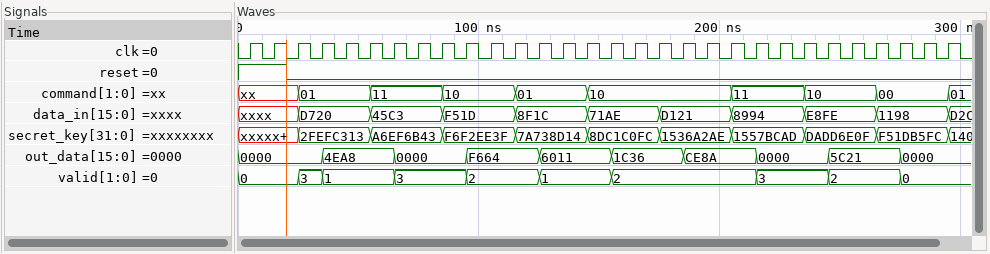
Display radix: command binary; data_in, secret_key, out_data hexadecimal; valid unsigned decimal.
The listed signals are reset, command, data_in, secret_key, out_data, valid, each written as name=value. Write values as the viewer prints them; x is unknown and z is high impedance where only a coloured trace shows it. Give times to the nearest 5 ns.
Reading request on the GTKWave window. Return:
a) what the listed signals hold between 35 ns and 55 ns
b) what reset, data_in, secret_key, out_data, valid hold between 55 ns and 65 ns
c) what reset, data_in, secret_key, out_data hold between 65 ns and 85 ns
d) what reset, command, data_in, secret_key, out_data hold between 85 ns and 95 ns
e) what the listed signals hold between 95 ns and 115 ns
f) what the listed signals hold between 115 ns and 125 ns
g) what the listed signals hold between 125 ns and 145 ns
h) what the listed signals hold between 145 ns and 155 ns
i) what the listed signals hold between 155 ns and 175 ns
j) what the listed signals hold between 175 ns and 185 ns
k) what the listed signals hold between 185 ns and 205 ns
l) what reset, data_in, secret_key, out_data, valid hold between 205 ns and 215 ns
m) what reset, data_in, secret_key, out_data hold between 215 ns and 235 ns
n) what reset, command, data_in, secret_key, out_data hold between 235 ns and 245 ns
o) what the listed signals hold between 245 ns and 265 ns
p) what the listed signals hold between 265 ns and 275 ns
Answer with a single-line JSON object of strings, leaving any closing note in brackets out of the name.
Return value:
{"what the listed signals hold between 35 ns and 55 ns": "reset=0, command=01, data_in=D720, secret_key=2FEFC313, out_data=4EA8, valid=1", "what reset, data_in, secret_key, out_data, valid hold between 55 ns and 65 ns": "reset=0, data_in=45C3, secret_key=A6EF6B43, out_data=4EA8, valid=1", "what reset, data_in, secret_key, out_data hold between 65 ns and 85 ns": "reset=0, data_in=45C3, secret_key=A6EF6B43, out_data=0000", "what reset, command, data_in, secret_key, out_data hold between 85 ns and 95 ns": "reset=0, command=10, data_in=F51D, secret_key=F6F2EE3F, out_data=0000", "what the listed signals hold between 95 ns and 115 ns": "reset=0, command=10, data_in=F51D, secret_key=F6F2EE3F, out_data=F664, valid=2", "what the listed signals hold between 115 ns and 125 ns": "reset=0, command=01, data_in=8F1C, secret_key=7A738D14, out_data=F664, valid=2", "what the listed signals hold between 125 ns and 145 ns": "reset=0, command=01, data_in=8F1C, secret_key=7A738D14, out_data=6011, valid=1", "what the listed signals hold between 145 ns and 155 ns": "reset=0, command=10, data_in=71AE, secret_key=8DC1C0FC, out_data=6011, valid=1", "what the listed signals hold between 155 ns and 175 ns": "reset=0, command=10, data_in=71AE, secret_key=8DC1C0FC, out_data=1C36, valid=2", "what the listed signals hold between 175 ns and 185 ns": "reset=0, command=10, data_in=D121, secret_key=1536A2AE, out_data=1C36, valid=2", "what the listed signals hold between 185 ns and 205 ns": "reset=0, command=10, data_in=D121, secret_key=1536A2AE, out_data=CE8A, valid=2", "what reset, data_in, secret_key, out_data, valid hold between 205 ns and 215 ns": "reset=0, data_in=8994, secret_key=1557BCAD, out_data=CE8A, valid=2", "what reset, data_in, secret_key, out_data hold between 215 ns and 235 ns": "reset=0, data_in=8994, secret_key=1557BCAD, out_data=0000", "what reset, command, data_in, secret_key, out_data hold between 235 ns and 245 ns": "reset=0, command=10, data_in=E8FE, secret_key=DADD6E0F, out_data=0000", "what the listed signals hold between 245 ns and 265 ns": "reset=0, command=10, data_in=E8FE, secret_key=DADD6E0F, out_data=5C21, valid=2", "what the listed signals hold between 265 ns and 275 ns": "reset=0, command=00, data_in=1198, secret_key=F51DB5FC, out_data=5C21, valid=2"}
